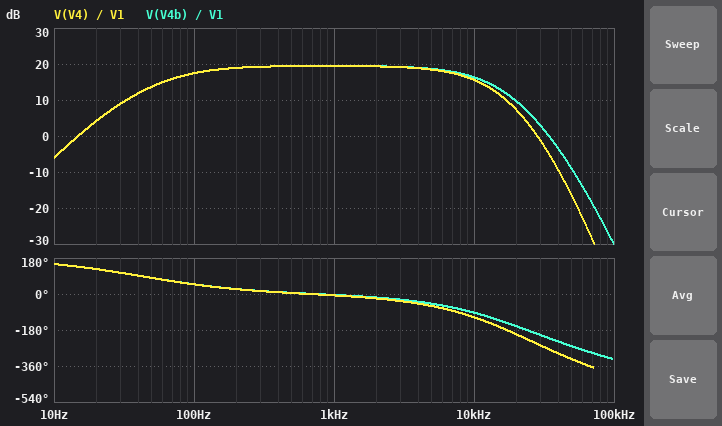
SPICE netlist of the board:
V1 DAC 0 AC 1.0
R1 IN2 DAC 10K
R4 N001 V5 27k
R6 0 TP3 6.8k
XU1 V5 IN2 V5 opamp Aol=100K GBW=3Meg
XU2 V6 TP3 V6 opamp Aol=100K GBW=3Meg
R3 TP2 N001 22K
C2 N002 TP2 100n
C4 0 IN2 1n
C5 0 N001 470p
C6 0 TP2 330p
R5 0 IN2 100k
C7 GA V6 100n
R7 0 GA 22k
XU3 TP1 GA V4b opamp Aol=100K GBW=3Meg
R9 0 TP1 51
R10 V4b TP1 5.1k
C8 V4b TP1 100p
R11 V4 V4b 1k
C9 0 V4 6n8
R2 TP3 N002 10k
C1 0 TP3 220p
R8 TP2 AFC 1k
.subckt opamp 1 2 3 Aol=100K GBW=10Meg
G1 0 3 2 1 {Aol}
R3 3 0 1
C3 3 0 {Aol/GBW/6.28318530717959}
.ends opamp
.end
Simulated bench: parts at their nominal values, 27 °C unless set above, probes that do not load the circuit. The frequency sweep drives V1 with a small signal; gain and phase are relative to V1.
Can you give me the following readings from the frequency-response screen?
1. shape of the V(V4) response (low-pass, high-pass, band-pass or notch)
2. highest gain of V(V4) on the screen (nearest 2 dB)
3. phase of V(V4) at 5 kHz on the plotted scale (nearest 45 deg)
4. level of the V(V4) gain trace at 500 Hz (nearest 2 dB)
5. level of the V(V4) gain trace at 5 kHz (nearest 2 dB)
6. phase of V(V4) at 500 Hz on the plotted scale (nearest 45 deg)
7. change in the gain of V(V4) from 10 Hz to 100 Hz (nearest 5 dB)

band-pass
20 dB
-45 deg
20 dB
18 dB
0 deg
25 dB
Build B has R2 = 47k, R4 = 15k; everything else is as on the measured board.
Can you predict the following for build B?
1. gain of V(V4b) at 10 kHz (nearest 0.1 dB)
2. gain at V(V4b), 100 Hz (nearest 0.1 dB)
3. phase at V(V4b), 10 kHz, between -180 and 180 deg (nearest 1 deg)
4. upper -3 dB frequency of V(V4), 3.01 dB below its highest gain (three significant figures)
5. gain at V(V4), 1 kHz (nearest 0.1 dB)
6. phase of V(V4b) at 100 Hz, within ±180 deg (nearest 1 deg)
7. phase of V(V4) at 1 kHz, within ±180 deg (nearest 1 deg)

13.3 dB
14.8 dB
-98 deg
8.43 kHz
16.7 dB
45 deg
-8 deg
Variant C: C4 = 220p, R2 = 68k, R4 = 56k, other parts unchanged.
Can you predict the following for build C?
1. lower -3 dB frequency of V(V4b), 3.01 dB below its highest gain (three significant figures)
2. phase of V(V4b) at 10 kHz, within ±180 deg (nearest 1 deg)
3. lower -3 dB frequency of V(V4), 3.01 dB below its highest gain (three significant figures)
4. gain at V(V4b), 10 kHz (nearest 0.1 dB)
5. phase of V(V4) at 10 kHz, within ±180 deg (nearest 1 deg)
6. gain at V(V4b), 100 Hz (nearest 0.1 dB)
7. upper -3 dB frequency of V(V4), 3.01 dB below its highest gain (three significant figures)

72.1 Hz
-103 deg
72.0 Hz
5.8 dB
-126 deg
10.3 dB
5.61 kHz
